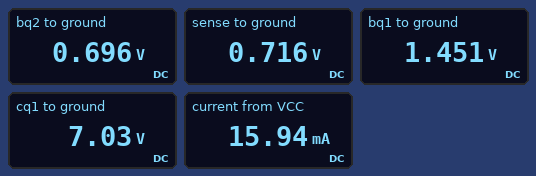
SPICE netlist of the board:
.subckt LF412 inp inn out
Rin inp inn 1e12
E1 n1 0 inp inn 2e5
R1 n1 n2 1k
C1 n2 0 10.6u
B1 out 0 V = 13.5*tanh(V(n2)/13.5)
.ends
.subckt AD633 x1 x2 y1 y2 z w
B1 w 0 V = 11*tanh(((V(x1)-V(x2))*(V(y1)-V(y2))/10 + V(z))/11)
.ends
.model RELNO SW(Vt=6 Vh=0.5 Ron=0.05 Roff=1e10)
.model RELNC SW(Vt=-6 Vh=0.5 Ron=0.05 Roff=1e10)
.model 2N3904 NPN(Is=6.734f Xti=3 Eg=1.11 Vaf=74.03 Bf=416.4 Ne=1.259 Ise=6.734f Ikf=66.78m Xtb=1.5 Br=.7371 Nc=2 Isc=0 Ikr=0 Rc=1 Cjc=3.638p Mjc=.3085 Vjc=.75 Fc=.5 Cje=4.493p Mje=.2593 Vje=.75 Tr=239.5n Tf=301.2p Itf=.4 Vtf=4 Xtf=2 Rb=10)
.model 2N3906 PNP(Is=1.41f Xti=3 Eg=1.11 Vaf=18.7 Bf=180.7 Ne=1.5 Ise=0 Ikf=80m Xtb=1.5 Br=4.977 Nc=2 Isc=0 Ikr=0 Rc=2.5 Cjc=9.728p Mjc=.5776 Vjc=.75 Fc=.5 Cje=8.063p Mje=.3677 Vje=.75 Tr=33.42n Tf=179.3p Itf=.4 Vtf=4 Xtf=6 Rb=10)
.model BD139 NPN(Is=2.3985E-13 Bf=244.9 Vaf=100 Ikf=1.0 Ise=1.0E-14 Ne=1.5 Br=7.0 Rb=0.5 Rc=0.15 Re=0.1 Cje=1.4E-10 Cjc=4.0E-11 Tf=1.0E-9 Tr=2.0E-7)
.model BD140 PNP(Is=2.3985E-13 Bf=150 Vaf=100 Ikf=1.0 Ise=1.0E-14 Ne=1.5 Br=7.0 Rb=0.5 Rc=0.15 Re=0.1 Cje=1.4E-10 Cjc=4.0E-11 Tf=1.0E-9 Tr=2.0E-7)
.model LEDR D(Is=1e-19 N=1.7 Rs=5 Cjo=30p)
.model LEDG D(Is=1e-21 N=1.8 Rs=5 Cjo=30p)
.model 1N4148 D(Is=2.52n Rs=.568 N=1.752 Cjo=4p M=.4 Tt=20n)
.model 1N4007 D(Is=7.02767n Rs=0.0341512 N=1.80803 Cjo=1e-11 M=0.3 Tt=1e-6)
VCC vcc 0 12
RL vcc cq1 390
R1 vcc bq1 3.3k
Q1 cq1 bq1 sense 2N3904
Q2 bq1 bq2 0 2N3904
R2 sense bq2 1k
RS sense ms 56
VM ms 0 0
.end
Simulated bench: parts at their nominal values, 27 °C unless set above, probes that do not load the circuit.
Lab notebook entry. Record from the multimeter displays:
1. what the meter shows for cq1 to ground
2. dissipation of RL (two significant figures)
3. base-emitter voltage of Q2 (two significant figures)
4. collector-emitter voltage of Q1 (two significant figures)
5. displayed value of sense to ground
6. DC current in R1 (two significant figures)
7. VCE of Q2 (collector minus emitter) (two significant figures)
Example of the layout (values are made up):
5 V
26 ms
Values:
7.03 V
63 mW
700 mV
6.3 V
0.716 V
3.2 mA
1.5 V
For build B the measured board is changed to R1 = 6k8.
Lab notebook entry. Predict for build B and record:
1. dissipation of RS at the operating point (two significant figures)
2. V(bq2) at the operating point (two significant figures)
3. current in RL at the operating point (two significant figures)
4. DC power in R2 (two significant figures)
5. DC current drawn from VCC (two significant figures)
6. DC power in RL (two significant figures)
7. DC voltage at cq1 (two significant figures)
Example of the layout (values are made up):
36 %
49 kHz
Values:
8.4 mW
680 mV
12 mA
110 nW
14 mA
58 mW
7.2 V
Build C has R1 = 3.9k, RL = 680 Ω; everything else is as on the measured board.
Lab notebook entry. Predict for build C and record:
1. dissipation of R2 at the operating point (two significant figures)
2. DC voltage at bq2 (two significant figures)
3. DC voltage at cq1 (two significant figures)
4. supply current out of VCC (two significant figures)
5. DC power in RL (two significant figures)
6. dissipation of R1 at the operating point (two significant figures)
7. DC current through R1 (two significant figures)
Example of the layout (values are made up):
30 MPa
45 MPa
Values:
310 nW
690 mV
3.4 V
15 mA
110 mW
29 mW
2.7 mA
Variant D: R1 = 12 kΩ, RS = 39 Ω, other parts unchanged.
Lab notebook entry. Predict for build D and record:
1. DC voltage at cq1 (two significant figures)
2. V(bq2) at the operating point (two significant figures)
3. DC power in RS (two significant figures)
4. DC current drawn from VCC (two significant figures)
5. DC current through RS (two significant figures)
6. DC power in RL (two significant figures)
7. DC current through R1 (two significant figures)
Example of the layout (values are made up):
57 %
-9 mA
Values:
5.4 V
660 mV
11 mW
18 mA
17 mA
110 mW
880 µA
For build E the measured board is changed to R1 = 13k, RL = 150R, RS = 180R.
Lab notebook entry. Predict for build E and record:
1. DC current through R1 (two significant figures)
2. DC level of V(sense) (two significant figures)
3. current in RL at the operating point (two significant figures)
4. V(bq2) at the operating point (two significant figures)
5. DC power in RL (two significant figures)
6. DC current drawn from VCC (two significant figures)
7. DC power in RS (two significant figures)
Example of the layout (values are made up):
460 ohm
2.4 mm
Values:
820 µA
670 mV
3.7 mA
660 mV
2.0 mW
4.5 mA
2.5 mW
